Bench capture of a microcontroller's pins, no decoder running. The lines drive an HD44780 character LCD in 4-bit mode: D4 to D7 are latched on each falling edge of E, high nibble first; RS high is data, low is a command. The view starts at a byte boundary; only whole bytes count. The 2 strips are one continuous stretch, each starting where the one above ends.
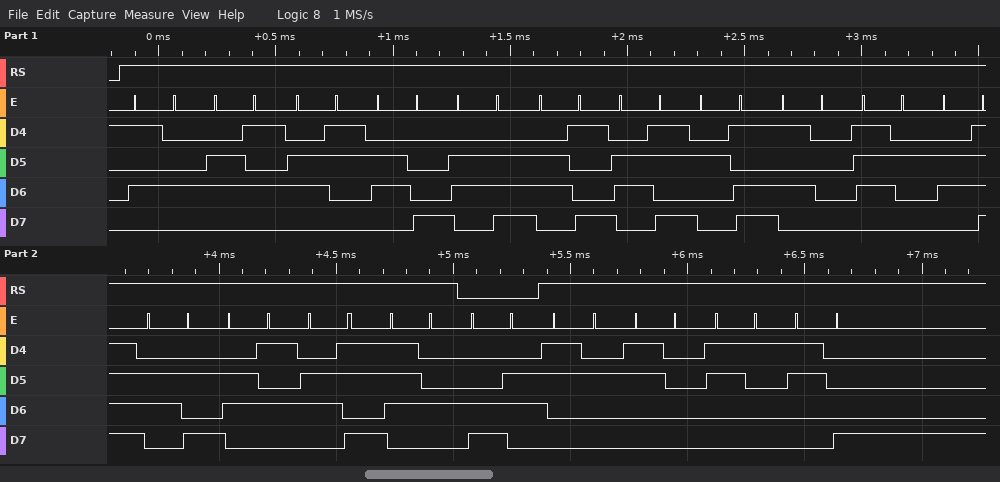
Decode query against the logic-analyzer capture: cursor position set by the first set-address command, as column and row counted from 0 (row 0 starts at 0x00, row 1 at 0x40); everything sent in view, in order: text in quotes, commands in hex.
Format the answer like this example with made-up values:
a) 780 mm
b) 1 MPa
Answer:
a) column 6, row 1
b) "Technik-Projekt" 0xC6 "2018"
